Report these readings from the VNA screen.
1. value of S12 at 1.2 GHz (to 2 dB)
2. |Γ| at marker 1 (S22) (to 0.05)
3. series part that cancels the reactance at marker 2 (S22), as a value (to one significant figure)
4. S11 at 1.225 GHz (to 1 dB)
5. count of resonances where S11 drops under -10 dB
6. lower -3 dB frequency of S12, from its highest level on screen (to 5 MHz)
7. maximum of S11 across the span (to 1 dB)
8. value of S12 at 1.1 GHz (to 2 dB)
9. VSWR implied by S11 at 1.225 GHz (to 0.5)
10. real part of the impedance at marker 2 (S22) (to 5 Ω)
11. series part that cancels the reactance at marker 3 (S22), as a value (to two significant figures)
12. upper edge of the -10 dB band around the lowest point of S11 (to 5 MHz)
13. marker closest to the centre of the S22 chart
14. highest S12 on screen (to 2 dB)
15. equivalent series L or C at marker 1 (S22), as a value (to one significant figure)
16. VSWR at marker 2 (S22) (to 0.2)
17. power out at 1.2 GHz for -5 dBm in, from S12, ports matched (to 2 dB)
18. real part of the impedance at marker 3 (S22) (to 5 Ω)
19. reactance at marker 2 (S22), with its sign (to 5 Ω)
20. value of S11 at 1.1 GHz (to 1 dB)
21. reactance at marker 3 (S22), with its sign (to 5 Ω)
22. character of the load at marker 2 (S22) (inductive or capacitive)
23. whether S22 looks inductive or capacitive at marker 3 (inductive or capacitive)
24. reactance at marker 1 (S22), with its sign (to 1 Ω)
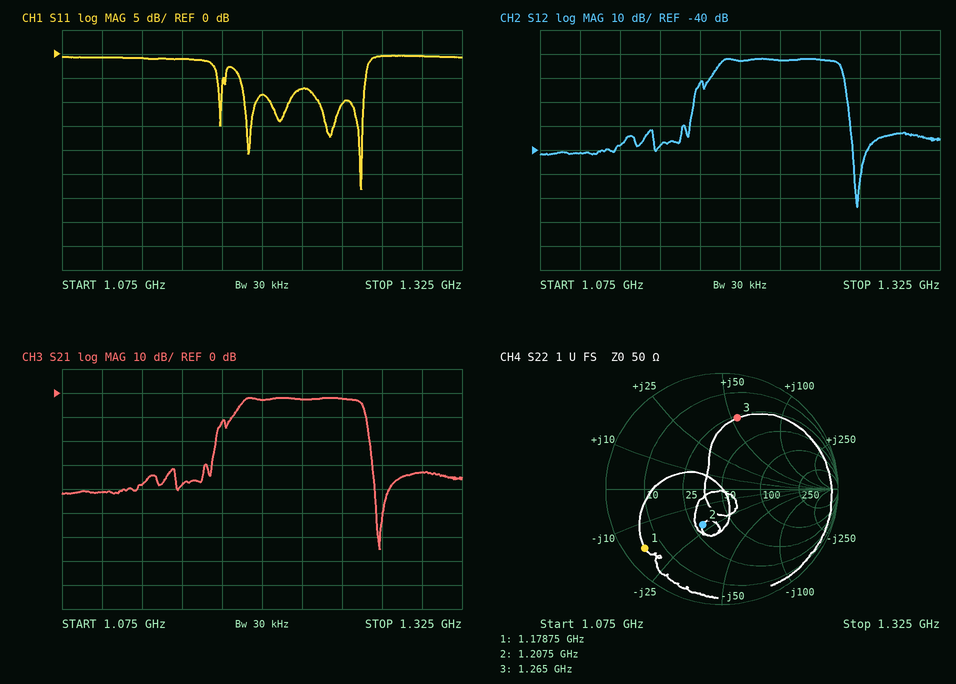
-2 dB
0.85
3 nH
-7 dB
5
1.185 GHz
0 dB
-42 dB
2.5
30 Ω
2.3 pF
1.265 GHz
marker 2
-2 dB
8 pF
2.0
-8 dBm
25 Ω
-20 Ω
-1 dB
+55 Ω
capacitive
inductive
-17 Ω
